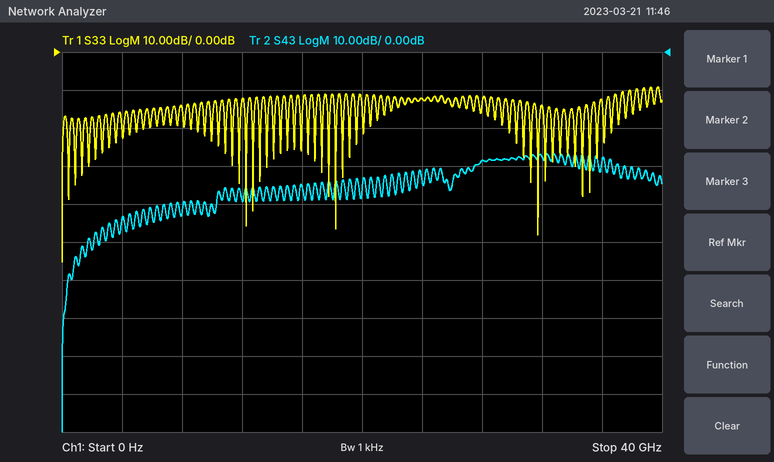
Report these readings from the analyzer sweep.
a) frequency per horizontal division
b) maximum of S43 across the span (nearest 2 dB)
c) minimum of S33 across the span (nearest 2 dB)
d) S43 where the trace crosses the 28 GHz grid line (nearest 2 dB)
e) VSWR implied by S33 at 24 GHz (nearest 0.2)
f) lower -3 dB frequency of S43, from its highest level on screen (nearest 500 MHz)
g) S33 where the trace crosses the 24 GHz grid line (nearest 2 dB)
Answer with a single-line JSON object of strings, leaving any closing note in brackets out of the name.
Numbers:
{"frequency per horizontal division": "4 GHz", "maximum of S43 across the span": "-26 dB", "minimum of S33 across the span": "-56 dB", "S43 where the trace crosses the 28 GHz grid line": "-28 dB", "VSWR implied by S33 at 24 GHz": "1.6", "lower -3 dB frequency of S43, from its highest level on screen": "27.5 GHz", "S33 where the trace crosses the 24 GHz grid line": "-12 dB"}
